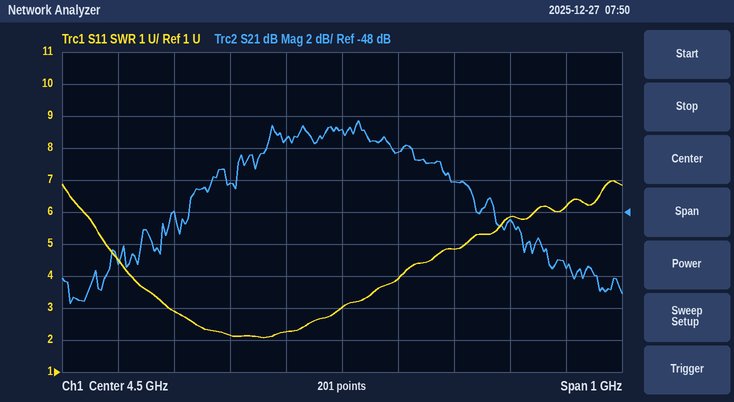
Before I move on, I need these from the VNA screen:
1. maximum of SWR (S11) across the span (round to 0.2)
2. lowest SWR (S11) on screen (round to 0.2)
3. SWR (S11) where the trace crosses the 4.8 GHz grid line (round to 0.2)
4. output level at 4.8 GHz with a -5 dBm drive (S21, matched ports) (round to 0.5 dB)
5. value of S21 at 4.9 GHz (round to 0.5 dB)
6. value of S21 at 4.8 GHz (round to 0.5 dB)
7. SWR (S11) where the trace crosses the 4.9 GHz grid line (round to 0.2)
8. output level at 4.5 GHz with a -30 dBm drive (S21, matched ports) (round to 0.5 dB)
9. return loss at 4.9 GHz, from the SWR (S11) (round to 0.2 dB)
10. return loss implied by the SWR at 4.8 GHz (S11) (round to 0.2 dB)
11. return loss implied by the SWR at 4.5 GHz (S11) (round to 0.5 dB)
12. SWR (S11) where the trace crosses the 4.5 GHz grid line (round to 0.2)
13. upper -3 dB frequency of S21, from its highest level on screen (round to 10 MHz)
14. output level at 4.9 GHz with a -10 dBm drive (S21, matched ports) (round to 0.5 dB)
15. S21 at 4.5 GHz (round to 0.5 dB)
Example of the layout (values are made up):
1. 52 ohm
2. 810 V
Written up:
1. 7.0
2. 2.0
3. 5.8
4. -53.5 dBm
5. -51.5 dB
6. -48.5 dB
7. 6.2
8. -73.0 dBm
9. 2.8 dB
10. 3.0 dB
11. 6.0 dB
12. 3.0
13. 4.68 GHz
14. -61.5 dBm
15. -43.0 dB
